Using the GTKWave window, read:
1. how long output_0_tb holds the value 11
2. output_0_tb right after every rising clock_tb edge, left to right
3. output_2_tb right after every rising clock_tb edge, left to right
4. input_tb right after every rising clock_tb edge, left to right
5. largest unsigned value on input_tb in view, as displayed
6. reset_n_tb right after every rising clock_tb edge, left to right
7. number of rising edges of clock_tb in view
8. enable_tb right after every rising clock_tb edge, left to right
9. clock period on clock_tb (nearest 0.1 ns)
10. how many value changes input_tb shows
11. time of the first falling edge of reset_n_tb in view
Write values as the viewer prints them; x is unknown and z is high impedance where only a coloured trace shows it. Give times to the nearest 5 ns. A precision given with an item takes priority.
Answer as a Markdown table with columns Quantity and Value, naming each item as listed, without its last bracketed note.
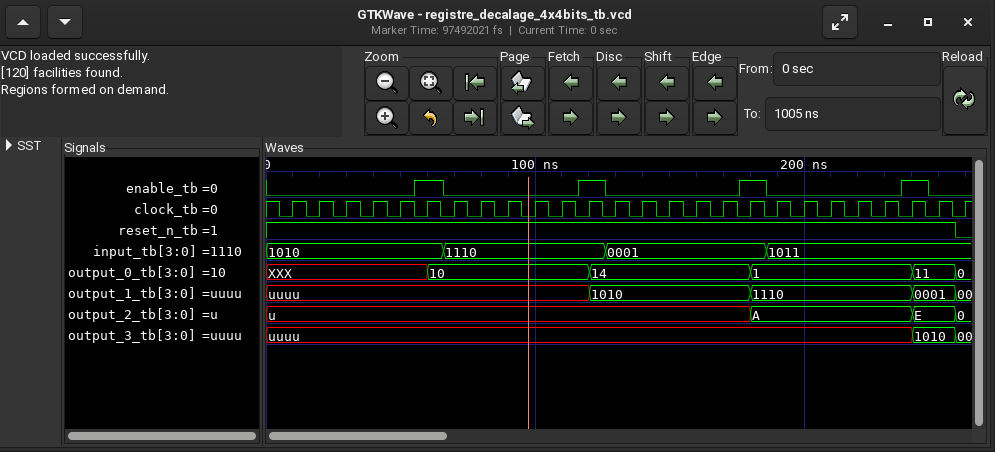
| Quantity | Value |
|---|---|
| how long output_0_tb holds the value 11 | 15 ns |
| output_0_tb right after every rising clock_tb edge, left to right | XXX, XXX, XXX, XXX, XXX, 10, 10, 10, 10, 10, 10, 14, 14, 14, 14, 14, 14, 1, 1, 1, 1, 1, 1, 11, 11, 0 |
| output_2_tb right after every rising clock_tb edge, left to right | u, u, u, u, u, u, u, u, u, u, u, u, u, u, u, u, u, A, A, A, A, A, A, E, E, 0 |
| input_tb right after every rising clock_tb edge, left to right | 1010, 1010, 1010, 1010, 1010, 1010, 1110, 1110, 1110, 1110, 1110, 1110, 0001, 0001, 0001, 0001, 0001, 0001, 1011, 1011, 1011, 1011, 1011, 1011, 1011, 1011 |
| largest unsigned value on input_tb in view, as displayed | 1110 |
| reset_n_tb right after every rising clock_tb edge, left to right | 1 1 1 1 1 1 1 1 1 1 1 1 1 1 1 1 1 1 1 1 1 1 1 1 1 0 |
| number of rising edges of clock_tb in view | 26 |
| enable_tb right after every rising clock_tb edge, left to right | 0 0 0 0 0 1 0 0 0 0 0 1 0 0 0 0 0 1 0 0 0 0 0 1 0 0 |
| clock period on clock_tb | 10 ns |
| how many value changes input_tb shows | 3 |
| time of the first falling edge of reset_n_tb in view | 255 ns |
